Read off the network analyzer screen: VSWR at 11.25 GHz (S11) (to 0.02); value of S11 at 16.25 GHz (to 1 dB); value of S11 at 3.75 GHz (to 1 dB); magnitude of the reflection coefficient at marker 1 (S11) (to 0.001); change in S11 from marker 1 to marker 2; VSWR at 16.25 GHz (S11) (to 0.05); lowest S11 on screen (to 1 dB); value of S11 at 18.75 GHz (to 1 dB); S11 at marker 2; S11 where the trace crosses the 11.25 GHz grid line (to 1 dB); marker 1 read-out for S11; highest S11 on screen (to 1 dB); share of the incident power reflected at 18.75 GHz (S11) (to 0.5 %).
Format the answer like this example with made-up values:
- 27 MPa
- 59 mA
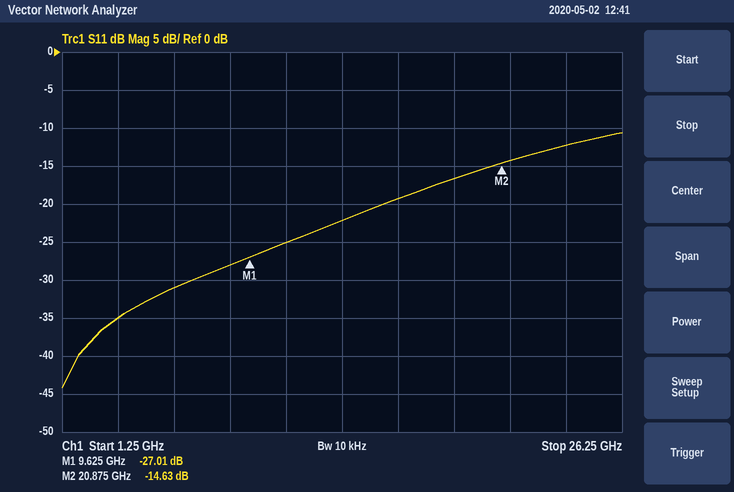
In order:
- 1.12
- -19 dB
- -35 dB
- 0.045
- 12.38 dB
- 1.25
- -44 dB
- -17 dB
- -14.63 dB
- -25 dB
- -27.01 dB
- -11 dB
- 2.0 %
